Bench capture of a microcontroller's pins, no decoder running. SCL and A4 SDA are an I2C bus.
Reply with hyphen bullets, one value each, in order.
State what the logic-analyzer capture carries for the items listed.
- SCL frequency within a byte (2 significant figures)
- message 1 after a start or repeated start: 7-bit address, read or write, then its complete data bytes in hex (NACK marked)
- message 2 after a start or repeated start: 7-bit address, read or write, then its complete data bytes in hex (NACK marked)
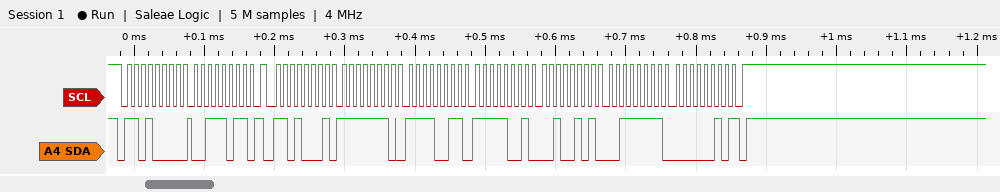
- 100 kHz
- 0x68 write: 3B
- 0x68 read: FE F3 F9 25 3F 02 NACK
